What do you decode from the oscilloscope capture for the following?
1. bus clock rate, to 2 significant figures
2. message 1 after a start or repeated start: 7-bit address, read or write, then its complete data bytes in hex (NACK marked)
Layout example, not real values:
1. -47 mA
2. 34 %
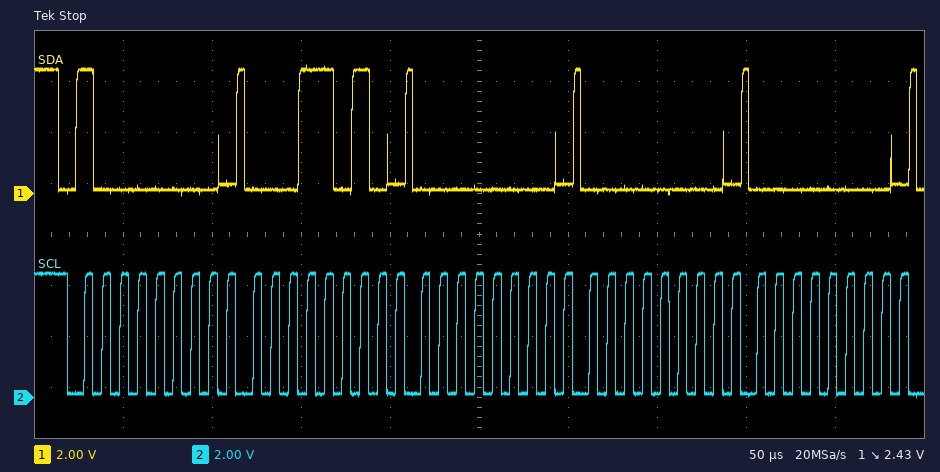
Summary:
1. 100 kHz
2. 0x40 write: 1A 00 00 00
